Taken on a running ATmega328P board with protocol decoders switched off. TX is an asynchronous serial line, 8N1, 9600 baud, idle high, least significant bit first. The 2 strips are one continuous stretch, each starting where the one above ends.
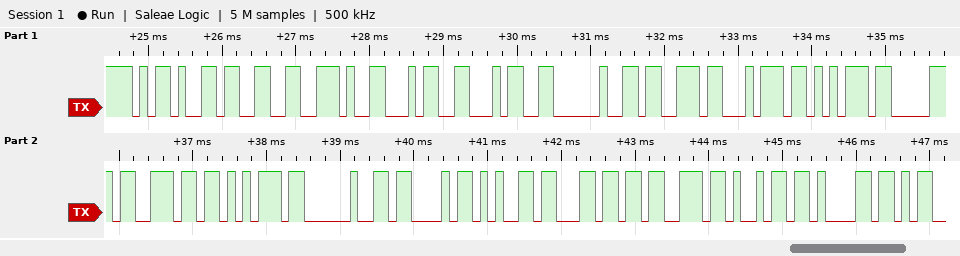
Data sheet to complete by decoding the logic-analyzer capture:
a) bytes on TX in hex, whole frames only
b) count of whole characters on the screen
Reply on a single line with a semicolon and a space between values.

0x2D 0x33 0x2E 0x34 0x34 0x20 0x73 0x74 0x75 0x70 0x6E 0x75 0x20 0x43 0x65 0x6C 0x73 0x69 0x61; 19
